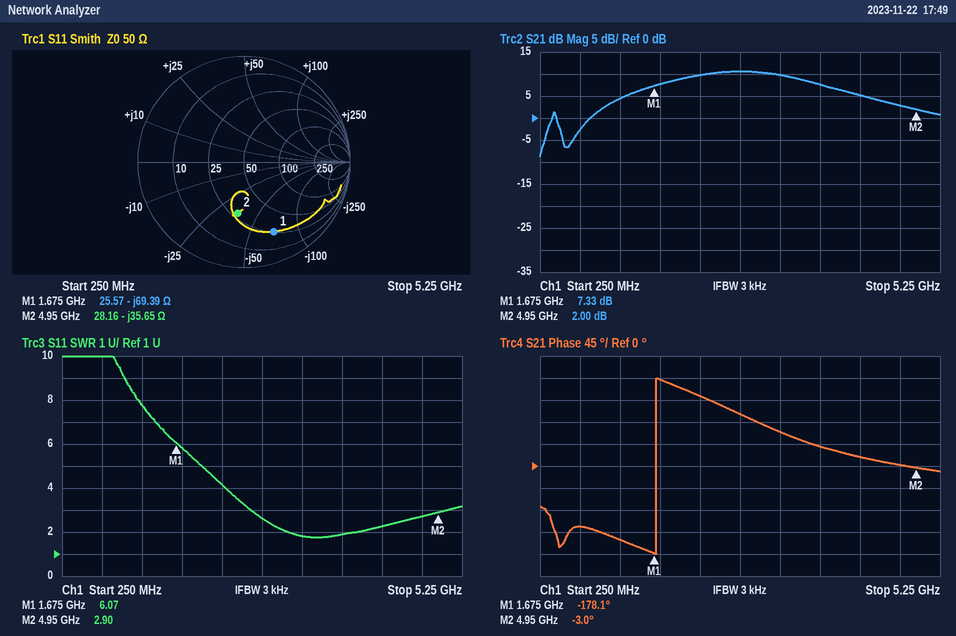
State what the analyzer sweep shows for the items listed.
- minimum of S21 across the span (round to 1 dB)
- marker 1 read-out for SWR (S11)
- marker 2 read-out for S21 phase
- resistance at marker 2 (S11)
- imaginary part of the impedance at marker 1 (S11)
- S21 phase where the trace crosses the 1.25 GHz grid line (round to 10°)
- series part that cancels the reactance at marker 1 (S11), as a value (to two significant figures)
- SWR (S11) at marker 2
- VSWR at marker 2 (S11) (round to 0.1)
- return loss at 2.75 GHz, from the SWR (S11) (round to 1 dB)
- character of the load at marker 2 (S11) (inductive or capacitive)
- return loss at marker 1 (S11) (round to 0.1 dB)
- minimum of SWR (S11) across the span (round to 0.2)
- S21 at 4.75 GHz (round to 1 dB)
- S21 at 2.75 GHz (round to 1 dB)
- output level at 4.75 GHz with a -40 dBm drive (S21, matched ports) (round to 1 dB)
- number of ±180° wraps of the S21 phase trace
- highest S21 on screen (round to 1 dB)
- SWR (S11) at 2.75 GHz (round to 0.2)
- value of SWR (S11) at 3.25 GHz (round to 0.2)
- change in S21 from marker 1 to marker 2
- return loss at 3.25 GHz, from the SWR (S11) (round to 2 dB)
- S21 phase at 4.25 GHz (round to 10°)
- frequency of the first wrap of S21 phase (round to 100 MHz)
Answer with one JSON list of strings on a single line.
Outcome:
["-9 dB", "6.07", "-3.0°", "28.16 Ω", "-69.39 Ω", "-150°", "6.6 nH", "2.90", "2.9", "7 dB", "capacitive", "2.9 dB", "1.8", "3 dB", "11 dB", "-37 dBm", "1", "11 dB", "2.6", "1.8", "-5.33 dB", "10 dB", "20°", "1.7 GHz"]
